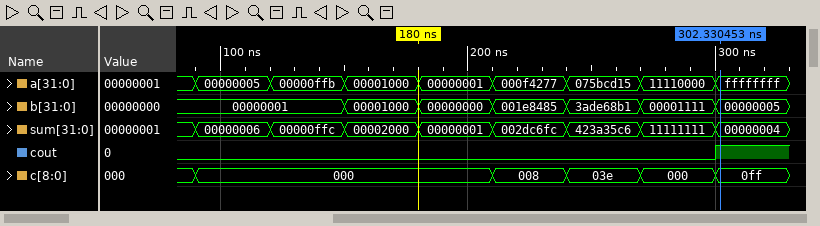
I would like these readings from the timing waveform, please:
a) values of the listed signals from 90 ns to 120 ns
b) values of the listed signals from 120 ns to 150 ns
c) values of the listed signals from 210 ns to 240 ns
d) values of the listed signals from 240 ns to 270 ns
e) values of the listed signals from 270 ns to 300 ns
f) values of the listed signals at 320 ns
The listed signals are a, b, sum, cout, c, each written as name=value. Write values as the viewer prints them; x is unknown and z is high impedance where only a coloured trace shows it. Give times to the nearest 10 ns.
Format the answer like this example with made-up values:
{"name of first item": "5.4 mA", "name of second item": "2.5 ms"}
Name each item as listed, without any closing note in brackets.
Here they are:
{"values of the listed signals from 90 ns to 120 ns": "a=00000005, b=00000001, sum=00000006, cout=0, c=000", "values of the listed signals from 120 ns to 150 ns": "a=00000ffb, b=00000001, sum=00000ffc, cout=0, c=000", "values of the listed signals from 210 ns to 240 ns": "a=000f4277, b=001e8485, sum=002dc6fc, cout=0, c=008", "values of the listed signals from 240 ns to 270 ns": "a=075bcd15, b=3ade68b1, sum=423a35c6, cout=0, c=03e", "values of the listed signals from 270 ns to 300 ns": "a=11110000, b=00001111, sum=11111111, cout=0, c=000", "values of the listed signals at 320 ns": "a=ffffffff, b=00000005, sum=00000004, cout=1, c=0ff"}
